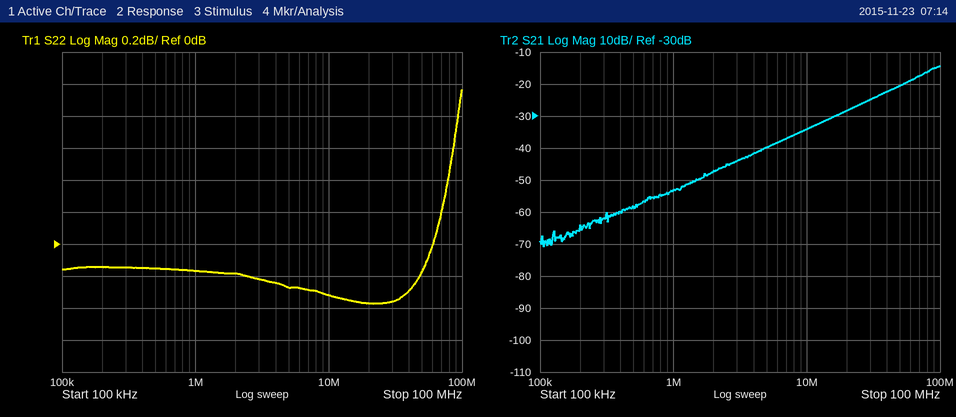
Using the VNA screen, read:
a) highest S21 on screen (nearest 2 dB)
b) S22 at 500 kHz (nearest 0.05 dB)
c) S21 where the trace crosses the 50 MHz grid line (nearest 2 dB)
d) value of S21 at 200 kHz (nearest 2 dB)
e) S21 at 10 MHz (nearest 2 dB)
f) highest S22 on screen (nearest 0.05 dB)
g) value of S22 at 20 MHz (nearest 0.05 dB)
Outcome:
-14 dB
-0.15 dB
-20 dB
-64 dB
-34 dB
0.95 dB
-0.35 dB
